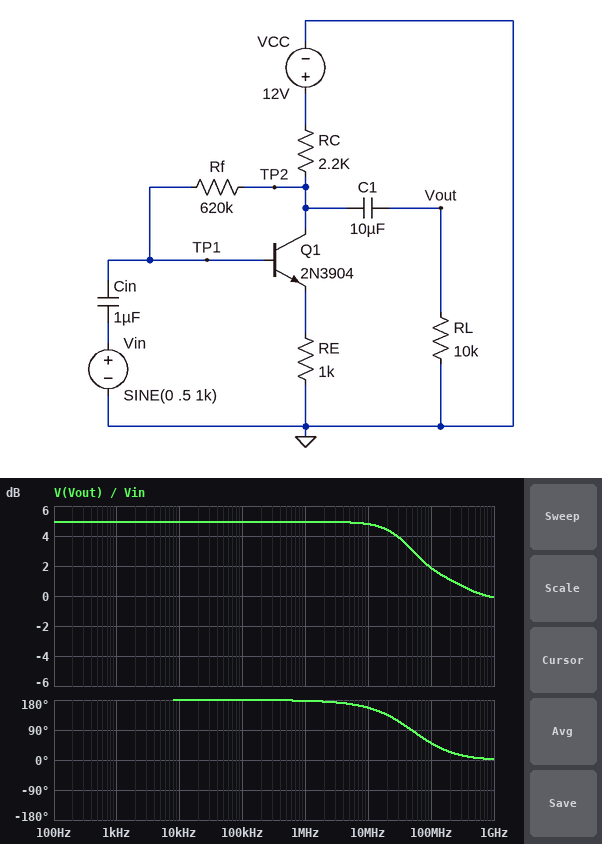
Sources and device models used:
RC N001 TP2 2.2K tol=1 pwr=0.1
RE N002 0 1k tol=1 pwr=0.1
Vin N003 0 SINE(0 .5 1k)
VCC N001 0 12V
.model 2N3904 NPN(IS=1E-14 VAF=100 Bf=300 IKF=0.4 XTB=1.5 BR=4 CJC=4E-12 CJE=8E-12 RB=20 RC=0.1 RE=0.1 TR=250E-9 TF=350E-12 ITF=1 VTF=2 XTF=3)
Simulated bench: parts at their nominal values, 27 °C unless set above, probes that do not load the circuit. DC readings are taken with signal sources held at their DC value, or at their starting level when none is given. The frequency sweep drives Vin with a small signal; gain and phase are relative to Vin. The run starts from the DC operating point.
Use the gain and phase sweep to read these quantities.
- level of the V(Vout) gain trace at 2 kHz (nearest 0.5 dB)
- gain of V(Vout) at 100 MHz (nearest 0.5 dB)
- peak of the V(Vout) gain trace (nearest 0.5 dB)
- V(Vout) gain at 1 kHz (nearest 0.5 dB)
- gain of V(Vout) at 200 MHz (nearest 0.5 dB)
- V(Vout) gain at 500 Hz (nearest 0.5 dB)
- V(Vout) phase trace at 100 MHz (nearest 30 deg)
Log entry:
5.0 dB
2.0 dB
5.0 dB
5.0 dB
1.0 dB
5.0 dB
60 deg
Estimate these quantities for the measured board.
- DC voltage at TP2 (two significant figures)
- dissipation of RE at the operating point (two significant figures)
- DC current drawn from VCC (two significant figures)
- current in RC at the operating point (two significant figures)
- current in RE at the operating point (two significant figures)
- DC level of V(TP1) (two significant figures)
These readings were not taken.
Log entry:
7.2 V
4.8 mW
2.2 mA
2.2 mA
2.2 mA
2.9 V
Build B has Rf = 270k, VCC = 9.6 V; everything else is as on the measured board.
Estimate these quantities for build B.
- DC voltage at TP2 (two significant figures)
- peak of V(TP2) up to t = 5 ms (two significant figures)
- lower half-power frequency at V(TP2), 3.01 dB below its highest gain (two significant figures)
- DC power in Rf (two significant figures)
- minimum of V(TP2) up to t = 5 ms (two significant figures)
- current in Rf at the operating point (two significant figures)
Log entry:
4.8 V
5.7 V
1.9 Hz
14 µW
3.9 V
7.2 µA
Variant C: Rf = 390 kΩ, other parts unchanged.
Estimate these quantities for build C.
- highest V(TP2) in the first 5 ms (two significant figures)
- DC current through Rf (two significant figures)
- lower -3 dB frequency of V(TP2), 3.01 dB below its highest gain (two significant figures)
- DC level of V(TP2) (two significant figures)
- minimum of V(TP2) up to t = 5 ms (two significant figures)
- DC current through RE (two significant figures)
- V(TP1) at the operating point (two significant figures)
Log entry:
7.3 V
8.2 µA
1.4 Hz
6.4 V
5.5 V
2.5 mA
3.2 V
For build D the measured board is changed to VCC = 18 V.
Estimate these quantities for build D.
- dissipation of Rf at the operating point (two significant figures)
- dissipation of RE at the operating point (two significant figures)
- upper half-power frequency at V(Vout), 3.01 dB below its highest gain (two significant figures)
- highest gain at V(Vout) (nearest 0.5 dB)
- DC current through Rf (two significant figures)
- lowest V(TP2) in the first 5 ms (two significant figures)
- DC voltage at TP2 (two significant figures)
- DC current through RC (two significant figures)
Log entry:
69 µW
11 mW
110 MHz
5.0 dB
11 µA
9.7 V
11 V
3.4 mA
